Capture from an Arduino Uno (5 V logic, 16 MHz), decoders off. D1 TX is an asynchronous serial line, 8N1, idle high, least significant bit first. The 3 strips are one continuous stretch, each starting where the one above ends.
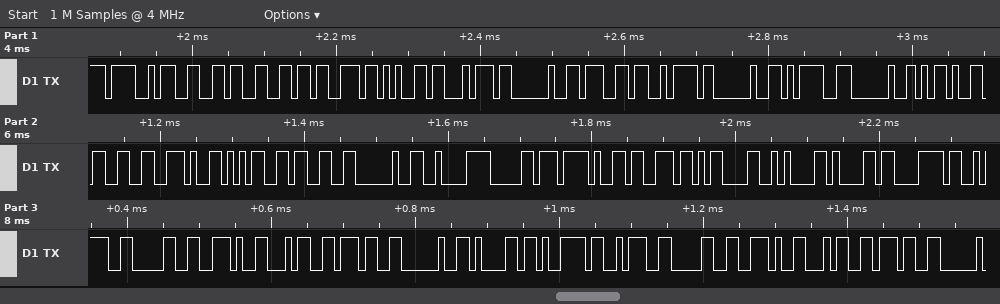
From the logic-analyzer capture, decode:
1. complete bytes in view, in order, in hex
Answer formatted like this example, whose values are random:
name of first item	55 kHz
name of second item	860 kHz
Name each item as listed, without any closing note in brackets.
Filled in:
complete bytes in view, in order, in hex	4F 66 66 73 65 74 20 67 7A 20 3D 20 2D 33 2E 35 33 20 C2 B0 2F 73 0D 0A 61 78 3A 30 2E 34 37 20 61 79 3A 30 2E 34 37
